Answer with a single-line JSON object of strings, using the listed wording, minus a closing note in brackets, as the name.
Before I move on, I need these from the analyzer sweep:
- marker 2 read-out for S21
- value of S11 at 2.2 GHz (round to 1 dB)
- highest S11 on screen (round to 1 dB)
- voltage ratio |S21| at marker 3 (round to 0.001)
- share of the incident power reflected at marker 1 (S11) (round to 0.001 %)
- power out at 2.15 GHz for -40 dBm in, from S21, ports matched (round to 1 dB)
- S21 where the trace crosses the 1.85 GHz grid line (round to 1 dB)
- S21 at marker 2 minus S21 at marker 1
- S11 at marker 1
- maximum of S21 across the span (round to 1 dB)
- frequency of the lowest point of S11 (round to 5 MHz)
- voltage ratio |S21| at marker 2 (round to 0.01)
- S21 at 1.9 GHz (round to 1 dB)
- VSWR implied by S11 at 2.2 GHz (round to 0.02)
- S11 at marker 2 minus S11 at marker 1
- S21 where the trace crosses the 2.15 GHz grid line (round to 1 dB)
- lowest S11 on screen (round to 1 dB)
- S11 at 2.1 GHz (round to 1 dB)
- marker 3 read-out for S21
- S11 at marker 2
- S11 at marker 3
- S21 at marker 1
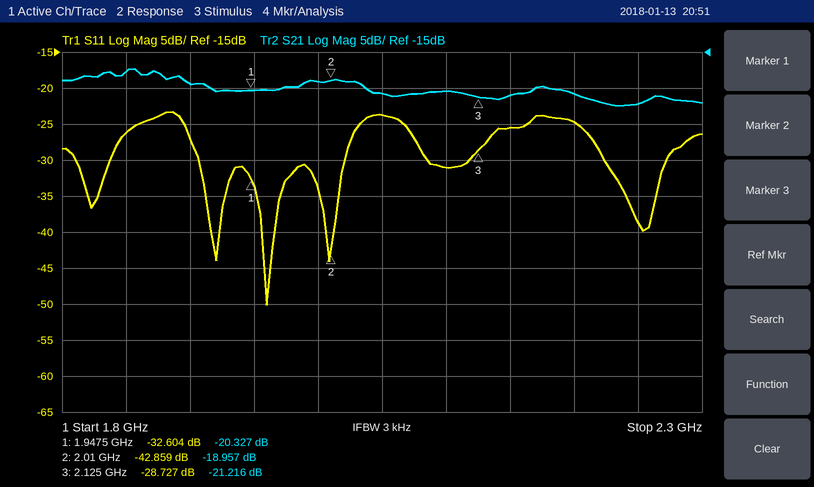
{"marker 2 read-out for S21": "-18.957 dB", "value of S11 at 2.2 GHz": "-25 dB", "highest S11 on screen": "-23 dB", "voltage ratio |S21| at marker 3": "0.087", "share of the incident power reflected at marker 1 (S11)": "0.055 %", "power out at 2.15 GHz for -40 dBm in, from S21, ports matched": "-61 dBm", "S21 where the trace crosses the 1.85 GHz grid line": "-18 dB", "S21 at marker 2 minus S21 at marker 1": "1.370 dB", "S11 at marker 1": "-32.604 dB", "maximum of S21 across the span": "-17 dB", "frequency of the lowest point of S11": "1.960 GHz", "voltage ratio |S21| at marker 2": "0.11", "S21 at 1.9 GHz": "-19 dB", "VSWR implied by S11 at 2.2 GHz": "1.12", "S11 at marker 2 minus S11 at marker 1": "-10.255 dB", "S21 where the trace crosses the 2.15 GHz grid line": "-21 dB", "lowest S11 on screen": "-50 dB", "S11 at 2.1 GHz": "-31 dB", "marker 3 read-out for S21": "-21.216 dB", "S11 at marker 2": "-42.859 dB", "S11 at marker 3": "-28.727 dB", "S21 at marker 1": "-20.327 dB"}
